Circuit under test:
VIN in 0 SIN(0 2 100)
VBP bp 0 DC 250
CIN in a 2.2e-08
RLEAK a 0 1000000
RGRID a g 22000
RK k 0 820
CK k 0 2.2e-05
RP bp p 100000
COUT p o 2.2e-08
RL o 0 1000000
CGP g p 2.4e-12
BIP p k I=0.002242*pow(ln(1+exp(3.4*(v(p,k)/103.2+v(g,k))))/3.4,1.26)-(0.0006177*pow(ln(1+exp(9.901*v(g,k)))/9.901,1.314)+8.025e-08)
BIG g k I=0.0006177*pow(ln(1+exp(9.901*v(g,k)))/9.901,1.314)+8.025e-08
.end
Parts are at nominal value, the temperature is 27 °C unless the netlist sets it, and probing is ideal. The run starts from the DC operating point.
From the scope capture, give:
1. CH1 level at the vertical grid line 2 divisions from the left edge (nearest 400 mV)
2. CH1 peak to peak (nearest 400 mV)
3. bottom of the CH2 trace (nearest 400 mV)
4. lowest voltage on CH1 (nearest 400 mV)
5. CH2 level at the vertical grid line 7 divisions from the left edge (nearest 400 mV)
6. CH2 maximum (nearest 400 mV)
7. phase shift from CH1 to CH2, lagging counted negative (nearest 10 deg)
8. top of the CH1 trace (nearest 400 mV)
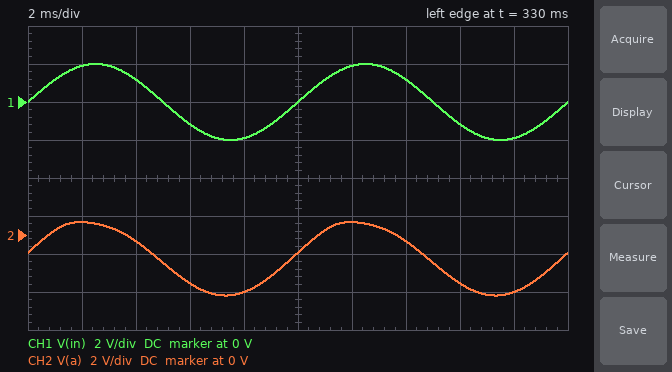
1.2 V
4.0 V
-3.2 V
-2.0 V
-400 mV
800 mV
10 deg
2.0 V
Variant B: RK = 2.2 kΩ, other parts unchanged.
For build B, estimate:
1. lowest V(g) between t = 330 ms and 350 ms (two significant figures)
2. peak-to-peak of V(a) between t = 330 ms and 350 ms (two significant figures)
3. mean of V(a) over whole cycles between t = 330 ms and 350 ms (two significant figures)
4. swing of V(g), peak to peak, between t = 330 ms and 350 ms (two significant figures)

-2.6 V
3.9 V
-600 mV
3.8 V
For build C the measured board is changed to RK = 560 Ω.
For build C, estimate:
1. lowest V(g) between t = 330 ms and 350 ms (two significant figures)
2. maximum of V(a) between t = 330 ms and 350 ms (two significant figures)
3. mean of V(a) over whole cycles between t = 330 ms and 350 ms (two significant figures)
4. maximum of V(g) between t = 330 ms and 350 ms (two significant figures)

-3.3 V
530 mV
-1.4 V
330 mV
